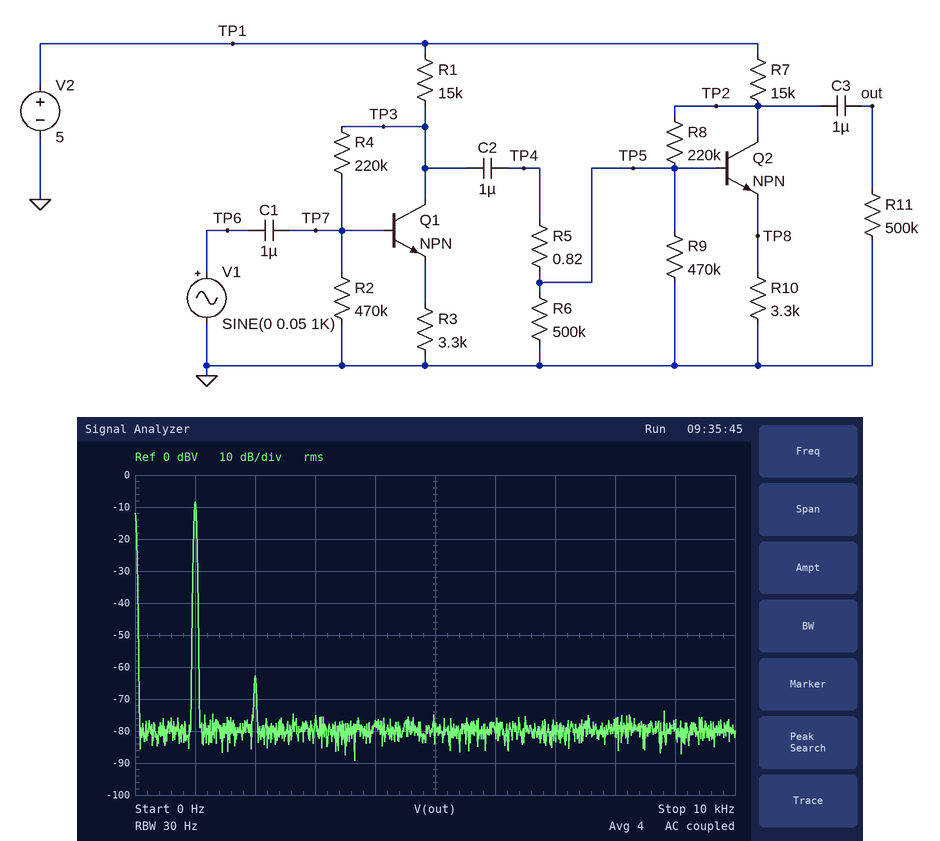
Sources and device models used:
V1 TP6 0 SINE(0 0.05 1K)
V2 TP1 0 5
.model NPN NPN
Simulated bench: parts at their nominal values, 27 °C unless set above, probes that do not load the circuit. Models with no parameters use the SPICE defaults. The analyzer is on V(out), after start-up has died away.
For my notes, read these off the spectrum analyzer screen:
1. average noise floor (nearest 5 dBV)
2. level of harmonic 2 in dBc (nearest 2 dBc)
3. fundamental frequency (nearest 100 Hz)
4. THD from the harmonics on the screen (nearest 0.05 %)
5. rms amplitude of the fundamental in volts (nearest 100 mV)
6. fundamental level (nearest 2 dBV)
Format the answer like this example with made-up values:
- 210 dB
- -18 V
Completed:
- -80 dBV
- -54 dBc
- 1.0 kHz
- 0.20 %
- 400 mV
- -8 dBV
